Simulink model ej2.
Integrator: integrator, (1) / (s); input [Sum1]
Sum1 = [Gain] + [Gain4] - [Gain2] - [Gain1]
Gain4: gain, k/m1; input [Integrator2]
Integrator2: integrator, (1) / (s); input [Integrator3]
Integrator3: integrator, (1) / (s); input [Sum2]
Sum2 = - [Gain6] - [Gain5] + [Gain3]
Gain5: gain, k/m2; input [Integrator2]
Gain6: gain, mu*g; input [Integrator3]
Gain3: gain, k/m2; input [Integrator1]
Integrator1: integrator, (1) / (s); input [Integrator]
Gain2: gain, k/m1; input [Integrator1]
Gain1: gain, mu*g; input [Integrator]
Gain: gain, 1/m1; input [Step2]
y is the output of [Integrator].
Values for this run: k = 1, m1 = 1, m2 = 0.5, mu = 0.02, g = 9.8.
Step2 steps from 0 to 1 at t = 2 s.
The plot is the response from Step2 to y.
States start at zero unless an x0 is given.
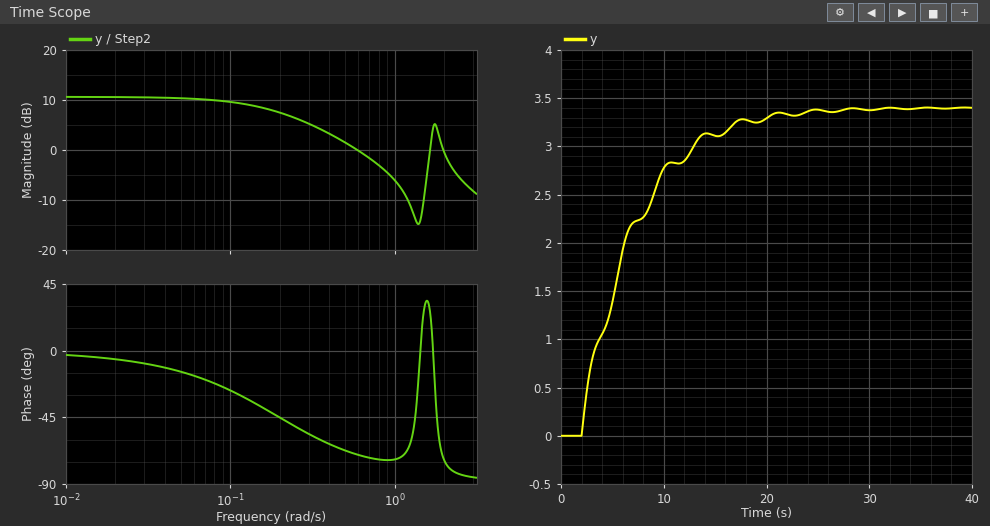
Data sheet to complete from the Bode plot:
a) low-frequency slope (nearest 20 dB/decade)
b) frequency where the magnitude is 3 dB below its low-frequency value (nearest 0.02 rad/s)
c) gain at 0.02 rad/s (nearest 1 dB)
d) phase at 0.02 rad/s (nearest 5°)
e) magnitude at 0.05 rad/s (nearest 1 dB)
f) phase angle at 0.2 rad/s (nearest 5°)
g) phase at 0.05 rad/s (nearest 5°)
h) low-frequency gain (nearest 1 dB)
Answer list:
0 dB/decade
0.20 rad/s
11 dB
-5°
10 dB
-45°
-15°
11 dB
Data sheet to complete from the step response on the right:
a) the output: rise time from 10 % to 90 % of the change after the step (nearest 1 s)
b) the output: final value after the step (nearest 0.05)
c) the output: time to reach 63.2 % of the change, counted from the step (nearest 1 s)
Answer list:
11 s
3.40
5 s
